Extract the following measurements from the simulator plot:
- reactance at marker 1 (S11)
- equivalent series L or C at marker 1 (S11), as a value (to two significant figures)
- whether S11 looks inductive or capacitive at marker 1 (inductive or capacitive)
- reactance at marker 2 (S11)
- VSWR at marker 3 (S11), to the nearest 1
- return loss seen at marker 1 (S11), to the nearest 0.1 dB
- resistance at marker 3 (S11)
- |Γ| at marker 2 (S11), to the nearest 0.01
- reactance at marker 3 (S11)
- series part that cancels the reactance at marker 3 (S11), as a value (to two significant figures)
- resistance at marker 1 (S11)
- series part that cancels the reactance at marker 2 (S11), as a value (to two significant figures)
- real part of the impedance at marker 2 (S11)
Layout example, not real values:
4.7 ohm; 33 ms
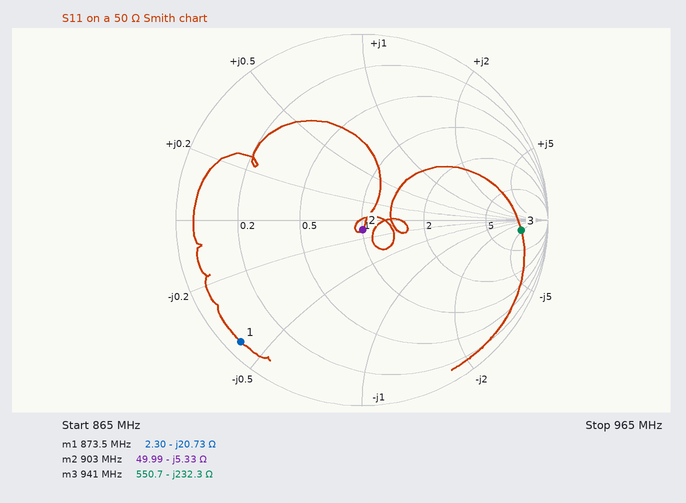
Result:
-20.73 Ω; 8.8 pF; capacitive; -5.33 Ω; 13; 0.7 dB; 550.7 Ω; 0.05; -232.3 Ω; 39 nH; 2.30 Ω; 940 pH; 49.99 Ω
